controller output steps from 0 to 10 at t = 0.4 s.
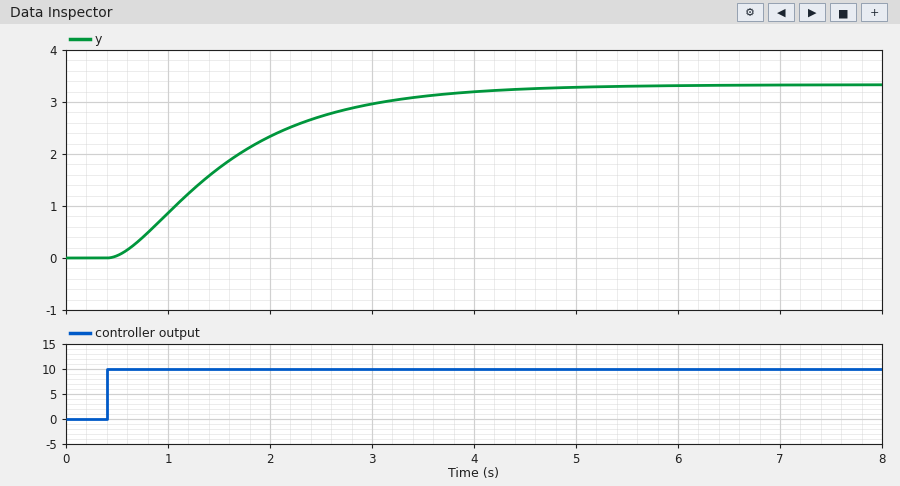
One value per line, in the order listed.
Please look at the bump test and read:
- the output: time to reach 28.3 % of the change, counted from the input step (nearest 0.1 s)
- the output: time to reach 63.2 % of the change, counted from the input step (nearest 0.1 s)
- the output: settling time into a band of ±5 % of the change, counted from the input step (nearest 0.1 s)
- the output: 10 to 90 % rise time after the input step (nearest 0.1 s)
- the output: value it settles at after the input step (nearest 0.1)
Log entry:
0.6 s
1.4 s
3.4 s
2.4 s
3.3
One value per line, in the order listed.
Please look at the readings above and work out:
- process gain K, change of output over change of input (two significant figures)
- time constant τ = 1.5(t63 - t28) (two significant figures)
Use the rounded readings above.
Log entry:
0.33
1.2 s
